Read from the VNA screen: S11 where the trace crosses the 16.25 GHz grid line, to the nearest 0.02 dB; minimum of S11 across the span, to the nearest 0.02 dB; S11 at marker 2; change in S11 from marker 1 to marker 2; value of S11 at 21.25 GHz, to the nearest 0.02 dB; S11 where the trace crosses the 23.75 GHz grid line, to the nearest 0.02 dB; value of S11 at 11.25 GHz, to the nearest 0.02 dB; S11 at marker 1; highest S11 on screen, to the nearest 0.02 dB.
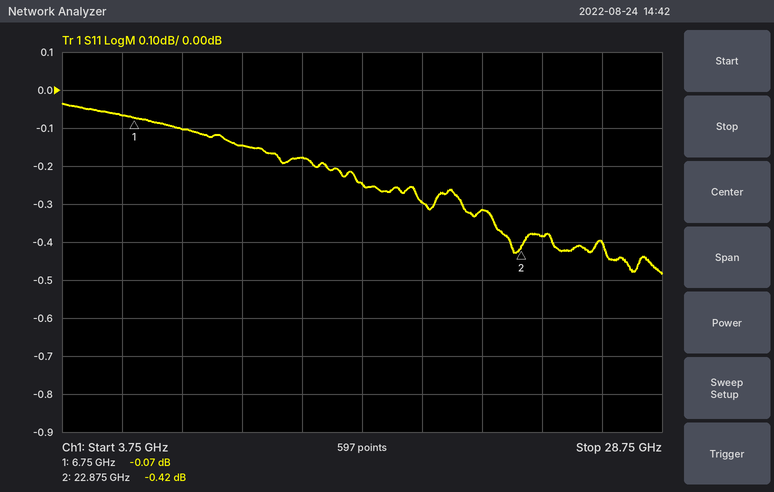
-0.24 dB
-0.48 dB
-0.42 dB
-0.35 dB
-0.32 dB
-0.38 dB
-0.14 dB
-0.07 dB
-0.04 dB
